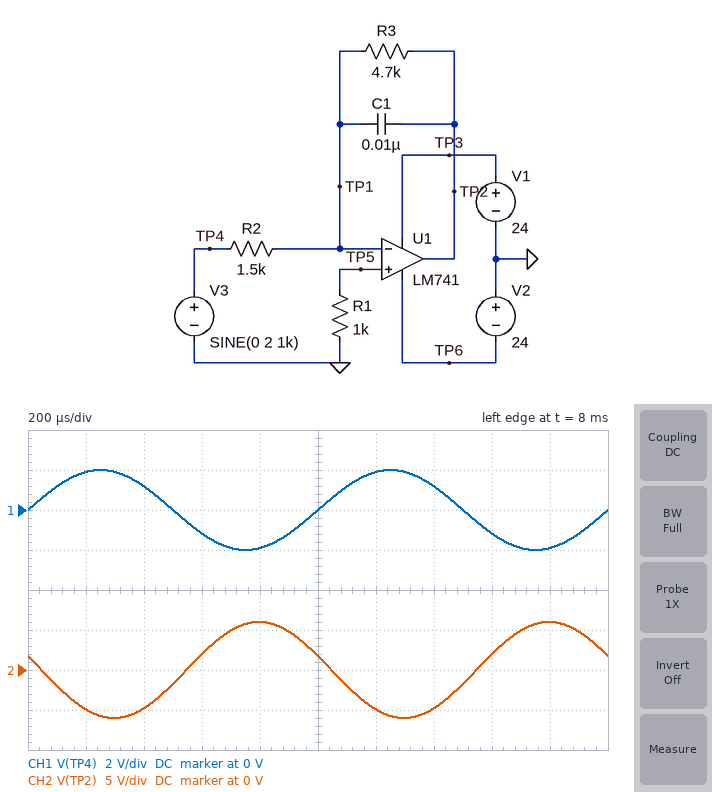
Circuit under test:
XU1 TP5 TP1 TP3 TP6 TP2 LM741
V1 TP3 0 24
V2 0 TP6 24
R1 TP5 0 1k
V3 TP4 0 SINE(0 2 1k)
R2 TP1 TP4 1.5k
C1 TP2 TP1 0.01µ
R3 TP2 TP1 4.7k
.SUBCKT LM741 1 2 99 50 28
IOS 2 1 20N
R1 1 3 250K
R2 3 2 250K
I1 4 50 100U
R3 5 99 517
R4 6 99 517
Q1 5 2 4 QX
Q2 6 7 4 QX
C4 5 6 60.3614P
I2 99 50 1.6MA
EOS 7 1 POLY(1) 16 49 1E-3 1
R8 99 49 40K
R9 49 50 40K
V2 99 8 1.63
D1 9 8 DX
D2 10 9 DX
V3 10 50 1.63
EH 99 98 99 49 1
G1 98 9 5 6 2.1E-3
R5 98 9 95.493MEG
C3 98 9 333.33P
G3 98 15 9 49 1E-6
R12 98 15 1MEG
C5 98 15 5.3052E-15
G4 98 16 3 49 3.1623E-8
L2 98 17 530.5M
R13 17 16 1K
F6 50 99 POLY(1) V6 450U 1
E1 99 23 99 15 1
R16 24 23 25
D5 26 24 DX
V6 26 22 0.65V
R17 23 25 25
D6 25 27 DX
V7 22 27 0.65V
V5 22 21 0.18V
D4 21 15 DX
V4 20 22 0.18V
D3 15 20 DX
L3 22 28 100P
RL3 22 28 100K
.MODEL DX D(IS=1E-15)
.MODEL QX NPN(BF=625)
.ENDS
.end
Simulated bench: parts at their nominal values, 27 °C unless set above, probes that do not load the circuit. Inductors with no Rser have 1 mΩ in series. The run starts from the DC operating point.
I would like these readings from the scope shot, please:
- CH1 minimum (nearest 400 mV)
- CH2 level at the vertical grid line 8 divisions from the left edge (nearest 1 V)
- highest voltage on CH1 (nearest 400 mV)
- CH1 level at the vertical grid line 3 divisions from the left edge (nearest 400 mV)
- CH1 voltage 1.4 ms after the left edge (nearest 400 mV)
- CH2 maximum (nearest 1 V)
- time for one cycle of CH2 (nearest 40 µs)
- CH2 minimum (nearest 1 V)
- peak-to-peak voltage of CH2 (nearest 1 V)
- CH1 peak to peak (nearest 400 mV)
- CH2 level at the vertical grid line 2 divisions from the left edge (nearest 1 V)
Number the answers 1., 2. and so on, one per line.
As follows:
1. -2.0 V
2. 2 V
3. 2.0 V
4. -1.2 V
5. 1.2 V
6. 6 V
7. 1.00 ms
8. -6 V
9. 12 V
10. 4.0 V
11. -5 V
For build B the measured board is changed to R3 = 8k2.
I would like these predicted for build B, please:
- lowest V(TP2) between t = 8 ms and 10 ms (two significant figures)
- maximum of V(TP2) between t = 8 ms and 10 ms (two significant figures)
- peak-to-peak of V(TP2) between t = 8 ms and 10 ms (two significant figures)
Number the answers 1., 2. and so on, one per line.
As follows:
1. -9.7 V
2. 9.7 V
3. 19 V
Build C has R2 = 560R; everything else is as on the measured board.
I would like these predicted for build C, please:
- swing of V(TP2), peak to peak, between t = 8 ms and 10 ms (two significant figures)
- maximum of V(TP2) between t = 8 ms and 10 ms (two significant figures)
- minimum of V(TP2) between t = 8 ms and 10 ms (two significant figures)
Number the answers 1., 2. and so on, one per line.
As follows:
1. 32 V
2. 16 V
3. -16 V
